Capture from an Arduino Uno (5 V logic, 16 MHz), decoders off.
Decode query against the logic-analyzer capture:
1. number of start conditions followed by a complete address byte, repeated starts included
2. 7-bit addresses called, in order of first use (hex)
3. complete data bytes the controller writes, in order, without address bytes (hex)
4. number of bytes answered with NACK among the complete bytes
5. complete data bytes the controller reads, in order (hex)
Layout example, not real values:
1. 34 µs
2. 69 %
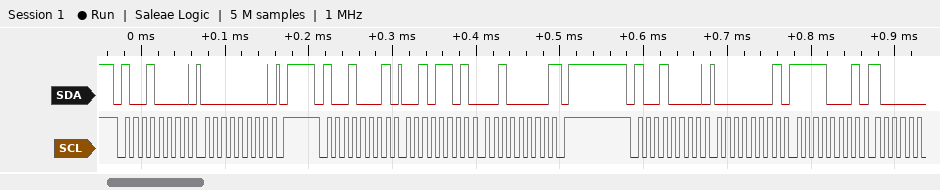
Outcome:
1. 3
2. 0x48
3. 00 01 F1
4. 1
5. 2D 20
